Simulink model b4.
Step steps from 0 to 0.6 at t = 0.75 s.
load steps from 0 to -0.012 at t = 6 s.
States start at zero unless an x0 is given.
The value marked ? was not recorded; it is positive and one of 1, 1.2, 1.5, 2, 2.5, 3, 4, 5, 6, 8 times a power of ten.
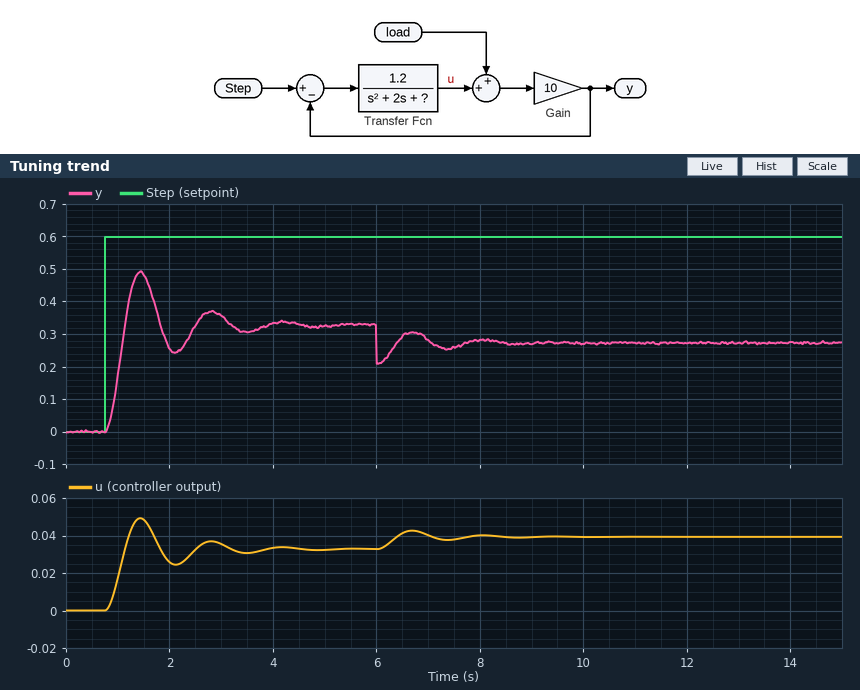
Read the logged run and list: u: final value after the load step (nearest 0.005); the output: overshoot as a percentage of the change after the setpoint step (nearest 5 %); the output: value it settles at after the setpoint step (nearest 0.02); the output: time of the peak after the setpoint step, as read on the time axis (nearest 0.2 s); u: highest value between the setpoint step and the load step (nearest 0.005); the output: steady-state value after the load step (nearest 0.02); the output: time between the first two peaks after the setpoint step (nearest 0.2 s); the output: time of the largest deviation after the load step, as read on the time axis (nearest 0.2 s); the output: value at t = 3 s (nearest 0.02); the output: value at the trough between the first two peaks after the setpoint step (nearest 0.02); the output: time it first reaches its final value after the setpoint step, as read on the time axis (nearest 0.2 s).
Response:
0.040
50 %
0.32
1.4 s
0.050
0.28
1.4 s
6.0 s
0.36
0.24
1.2 s
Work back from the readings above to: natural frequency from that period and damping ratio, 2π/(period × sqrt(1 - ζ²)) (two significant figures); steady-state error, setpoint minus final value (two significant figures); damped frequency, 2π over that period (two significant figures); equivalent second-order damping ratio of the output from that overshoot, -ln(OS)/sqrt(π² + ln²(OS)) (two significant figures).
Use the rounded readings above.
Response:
4.6 rad/s
0.28
4.5 rad/s
0.22
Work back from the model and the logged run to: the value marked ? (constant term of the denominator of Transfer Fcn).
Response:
10
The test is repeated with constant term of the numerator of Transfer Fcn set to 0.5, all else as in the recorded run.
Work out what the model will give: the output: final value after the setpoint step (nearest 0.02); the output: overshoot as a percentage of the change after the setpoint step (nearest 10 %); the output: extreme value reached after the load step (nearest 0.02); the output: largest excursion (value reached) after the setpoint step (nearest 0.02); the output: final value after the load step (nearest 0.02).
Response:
0.20
40 %
0.08
0.28
0.12
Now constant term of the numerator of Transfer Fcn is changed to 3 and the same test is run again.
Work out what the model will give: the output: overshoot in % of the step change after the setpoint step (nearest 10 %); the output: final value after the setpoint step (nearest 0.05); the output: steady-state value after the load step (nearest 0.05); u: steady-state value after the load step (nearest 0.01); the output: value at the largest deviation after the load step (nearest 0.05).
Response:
60 %
0.45
0.40
0.05
0.35
